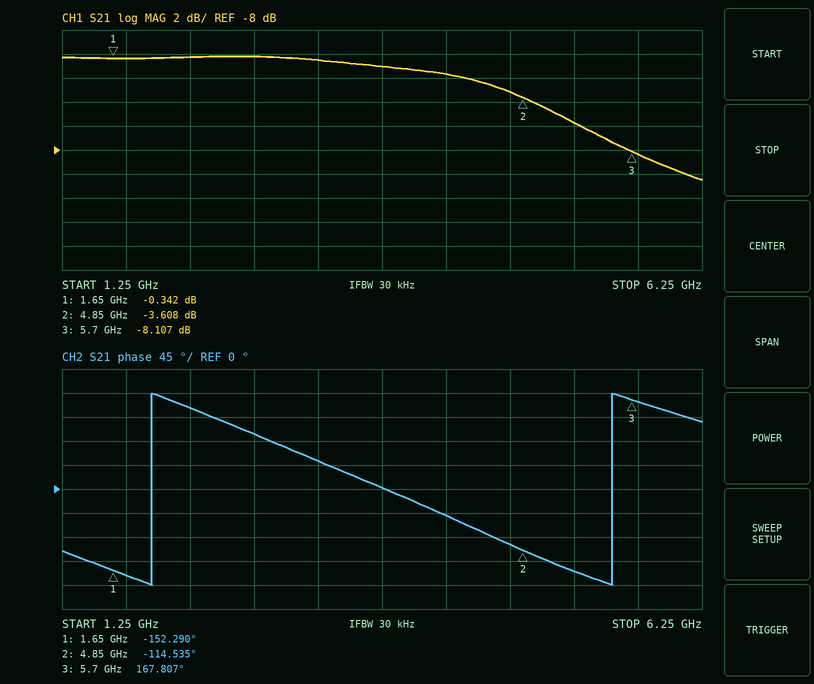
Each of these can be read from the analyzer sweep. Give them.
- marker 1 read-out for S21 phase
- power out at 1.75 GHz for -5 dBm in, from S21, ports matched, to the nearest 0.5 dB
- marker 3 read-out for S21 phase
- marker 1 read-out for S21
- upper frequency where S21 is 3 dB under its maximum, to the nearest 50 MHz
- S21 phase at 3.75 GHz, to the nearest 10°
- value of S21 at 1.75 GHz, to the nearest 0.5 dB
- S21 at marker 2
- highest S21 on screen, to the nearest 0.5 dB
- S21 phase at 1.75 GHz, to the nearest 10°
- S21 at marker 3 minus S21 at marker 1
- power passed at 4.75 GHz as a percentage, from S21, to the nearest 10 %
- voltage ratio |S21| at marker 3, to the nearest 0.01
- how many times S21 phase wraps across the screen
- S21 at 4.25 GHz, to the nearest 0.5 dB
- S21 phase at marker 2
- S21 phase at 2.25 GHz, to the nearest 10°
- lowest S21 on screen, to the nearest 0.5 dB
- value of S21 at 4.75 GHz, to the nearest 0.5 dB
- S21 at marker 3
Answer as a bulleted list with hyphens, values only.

- -152.290°
- -5.5 dBm
- 167.807°
- -0.342 dB
- 4.75 GHz
- 0°
- -0.5 dB
- -3.608 dB
- 0.0 dB
- -160°
- -7.765 dB
- 50 %
- 0.39
- 2
- -1.5 dB
- -114.535°
- 150°
- -10.5 dB
- -3.0 dB
- -8.107 dB
